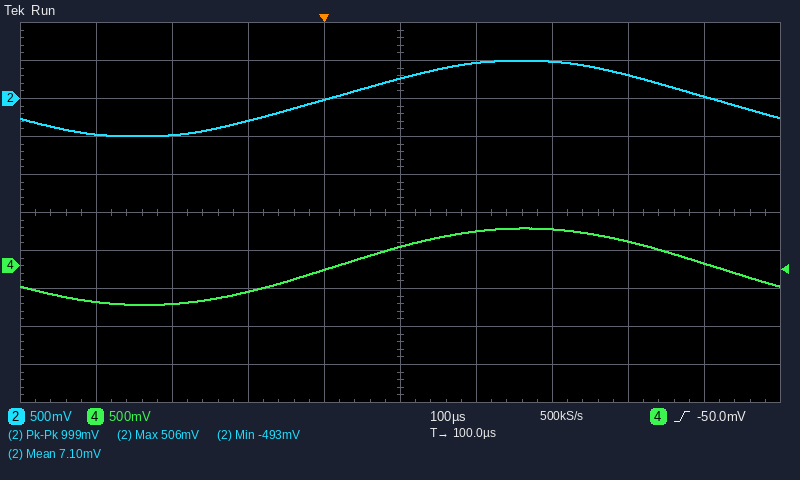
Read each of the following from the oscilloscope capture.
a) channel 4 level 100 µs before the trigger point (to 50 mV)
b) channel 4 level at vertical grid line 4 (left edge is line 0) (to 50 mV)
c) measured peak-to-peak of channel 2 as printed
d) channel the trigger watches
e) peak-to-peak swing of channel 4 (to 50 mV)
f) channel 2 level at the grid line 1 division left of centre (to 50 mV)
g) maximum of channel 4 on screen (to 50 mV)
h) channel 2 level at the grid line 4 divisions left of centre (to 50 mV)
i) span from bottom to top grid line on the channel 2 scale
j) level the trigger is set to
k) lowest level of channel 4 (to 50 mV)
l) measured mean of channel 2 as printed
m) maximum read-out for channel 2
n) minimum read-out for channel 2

-350 mV
-50 mV
999 mV
channel 4
1.00 V
0 mV
500 mV
-450 mV
5 V
-50.0 mV
-500 mV
7.10 mV
506 mV
-493 mV
